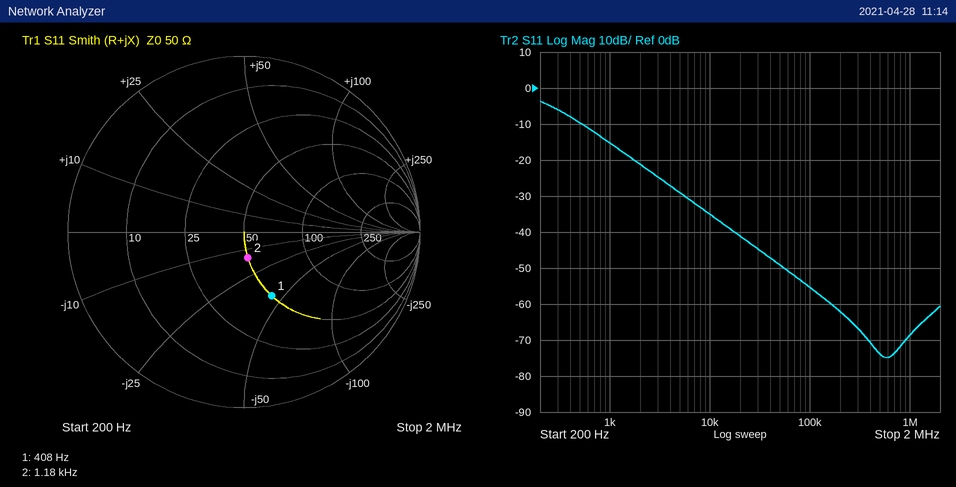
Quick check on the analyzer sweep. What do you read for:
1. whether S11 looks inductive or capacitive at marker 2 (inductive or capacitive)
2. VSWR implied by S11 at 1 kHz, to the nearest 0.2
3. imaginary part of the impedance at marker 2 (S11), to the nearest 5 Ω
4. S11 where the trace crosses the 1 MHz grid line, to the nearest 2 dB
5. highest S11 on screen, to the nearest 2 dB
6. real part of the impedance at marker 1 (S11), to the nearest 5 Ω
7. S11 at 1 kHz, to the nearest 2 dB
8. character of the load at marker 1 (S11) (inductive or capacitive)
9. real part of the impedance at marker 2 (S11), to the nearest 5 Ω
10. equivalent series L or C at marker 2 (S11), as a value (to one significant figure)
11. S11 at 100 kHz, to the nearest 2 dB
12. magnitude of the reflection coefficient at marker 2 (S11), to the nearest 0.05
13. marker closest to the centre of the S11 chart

capacitive
1.4
-15 Ω
-68 dB
-4 dB
50 Ω
-16 dB
capacitive
50 Ω
9 µF
-56 dB
0.15
marker 2
